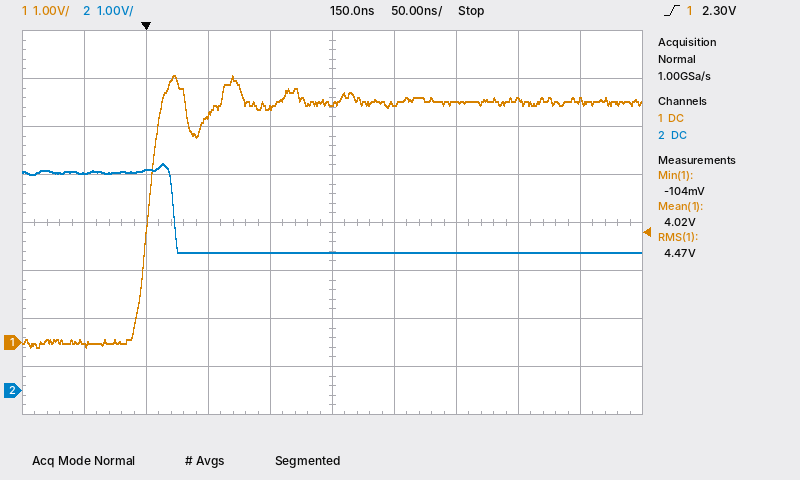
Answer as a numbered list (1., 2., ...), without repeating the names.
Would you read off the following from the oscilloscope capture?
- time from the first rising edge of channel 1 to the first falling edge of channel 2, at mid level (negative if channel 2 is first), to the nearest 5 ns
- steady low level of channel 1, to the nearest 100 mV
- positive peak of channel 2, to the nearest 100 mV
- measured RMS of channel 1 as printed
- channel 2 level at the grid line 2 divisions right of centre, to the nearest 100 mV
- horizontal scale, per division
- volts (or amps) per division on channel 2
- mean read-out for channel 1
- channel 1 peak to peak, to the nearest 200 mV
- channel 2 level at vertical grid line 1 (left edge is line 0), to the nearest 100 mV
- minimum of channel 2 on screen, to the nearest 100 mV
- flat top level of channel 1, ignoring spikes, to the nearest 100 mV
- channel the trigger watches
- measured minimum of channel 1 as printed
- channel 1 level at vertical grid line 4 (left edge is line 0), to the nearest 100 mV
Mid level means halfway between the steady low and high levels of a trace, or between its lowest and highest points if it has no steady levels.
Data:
1. +20 ns
2. 0.0 V
3. 4.7 V
4. 4.47 V
5. 2.9 V
6. 50 ns
7. 1 V
8. 4.02 V
9. 5.6 V
10. 4.5 V
11. 2.9 V
12. 5.0 V
13. channel 1
14. -104 mV
15. 4.9 V
